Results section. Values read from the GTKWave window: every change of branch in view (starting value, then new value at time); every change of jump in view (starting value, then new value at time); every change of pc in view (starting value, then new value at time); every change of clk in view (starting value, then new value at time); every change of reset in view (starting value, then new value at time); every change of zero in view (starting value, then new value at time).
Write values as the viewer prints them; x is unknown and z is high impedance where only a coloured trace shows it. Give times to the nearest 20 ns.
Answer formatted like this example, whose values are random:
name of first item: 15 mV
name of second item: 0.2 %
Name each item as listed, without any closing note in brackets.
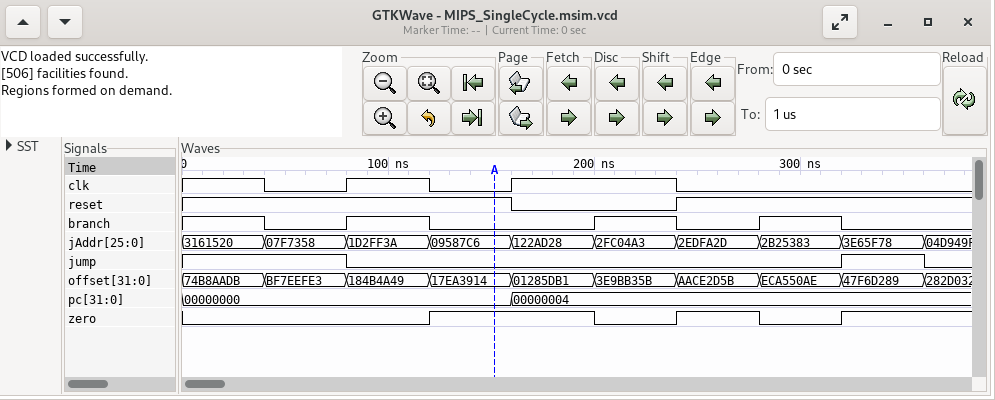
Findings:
every change of branch in view: 1, 0 at 40 ns, 1 at 80 ns, 0 at 120 ns, 1 at 200 ns, 0 at 240 ns, 1 at 280 ns, 0 at 320 ns
every change of jump in view: 1, 0 at 80 ns, 1 at 320 ns, 0 at 360 ns
every change of pc in view: 00000000, 00000004 at 160 ns
every change of clk in view: 1, 0 at 40 ns, 1 at 80 ns, 0 at 120 ns, 1 at 160 ns, 0 at 240 ns
every change of reset in view: 1, 0 at 160 ns, 1 at 240 ns
every change of zero in view: 0, 1 at 120 ns, 0 at 200 ns, 1 at 240 ns, 0 at 280 ns, 1 at 320 ns
